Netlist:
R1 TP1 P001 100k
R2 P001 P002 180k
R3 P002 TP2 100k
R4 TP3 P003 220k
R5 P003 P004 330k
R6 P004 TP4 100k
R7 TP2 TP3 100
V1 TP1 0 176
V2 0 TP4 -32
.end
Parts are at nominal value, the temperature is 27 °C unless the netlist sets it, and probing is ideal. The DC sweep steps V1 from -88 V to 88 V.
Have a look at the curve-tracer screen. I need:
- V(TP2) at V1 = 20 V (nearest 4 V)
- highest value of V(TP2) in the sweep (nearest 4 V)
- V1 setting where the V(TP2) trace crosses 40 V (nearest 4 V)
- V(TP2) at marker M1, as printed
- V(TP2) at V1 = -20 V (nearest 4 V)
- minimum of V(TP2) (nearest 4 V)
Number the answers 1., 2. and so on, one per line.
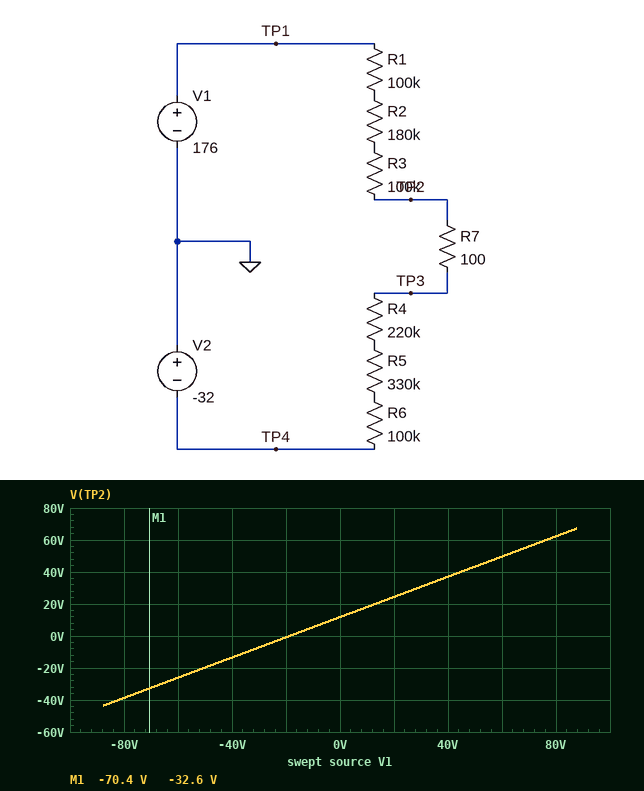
1. 24 V
2. 68 V
3. 44 V
4. -32.6 V
5. 0 V
6. -44 V
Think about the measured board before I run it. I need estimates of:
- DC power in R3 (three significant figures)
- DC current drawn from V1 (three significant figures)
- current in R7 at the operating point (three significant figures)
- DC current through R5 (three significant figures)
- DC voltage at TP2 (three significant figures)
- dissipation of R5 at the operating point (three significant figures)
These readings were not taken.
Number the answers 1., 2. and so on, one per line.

1. 1.95 mW
2. 140 µA
3. 140 µA
4. 140 µA
5. 123 V
6. 6.45 mW
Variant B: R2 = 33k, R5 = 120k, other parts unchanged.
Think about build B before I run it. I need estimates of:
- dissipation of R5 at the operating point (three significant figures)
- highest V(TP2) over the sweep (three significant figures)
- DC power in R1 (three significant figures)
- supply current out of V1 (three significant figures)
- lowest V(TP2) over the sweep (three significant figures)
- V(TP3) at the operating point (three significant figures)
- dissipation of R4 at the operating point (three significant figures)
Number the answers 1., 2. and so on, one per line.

1. 5.49 mW
2. 68.6 V
3. 4.58 mW
4. 214 µA
5. -46.5 V
6. 126 V
7. 10.1 mW
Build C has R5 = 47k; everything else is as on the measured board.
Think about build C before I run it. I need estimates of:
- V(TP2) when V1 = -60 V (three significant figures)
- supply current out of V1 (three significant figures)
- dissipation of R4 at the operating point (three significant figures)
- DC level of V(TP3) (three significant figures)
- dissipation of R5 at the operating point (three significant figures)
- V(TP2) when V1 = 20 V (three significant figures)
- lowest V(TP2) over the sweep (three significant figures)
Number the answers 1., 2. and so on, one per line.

1. -13.2 V
2. 193 µA
3. 8.17 mW
4. 103 V
5. 1.75 mW
6. 26.1 V
7. -27.0 V
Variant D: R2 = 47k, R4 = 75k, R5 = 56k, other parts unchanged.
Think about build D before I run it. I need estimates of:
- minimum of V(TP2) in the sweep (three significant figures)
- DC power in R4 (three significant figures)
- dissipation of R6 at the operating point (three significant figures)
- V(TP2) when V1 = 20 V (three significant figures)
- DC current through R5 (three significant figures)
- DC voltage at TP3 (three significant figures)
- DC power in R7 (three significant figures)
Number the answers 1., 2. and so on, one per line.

1. -26.0 V
2. 6.80 mW
3. 9.07 mW
4. 26.2 V
5. 301 µA
6. 102 V
7. 9.07 µW
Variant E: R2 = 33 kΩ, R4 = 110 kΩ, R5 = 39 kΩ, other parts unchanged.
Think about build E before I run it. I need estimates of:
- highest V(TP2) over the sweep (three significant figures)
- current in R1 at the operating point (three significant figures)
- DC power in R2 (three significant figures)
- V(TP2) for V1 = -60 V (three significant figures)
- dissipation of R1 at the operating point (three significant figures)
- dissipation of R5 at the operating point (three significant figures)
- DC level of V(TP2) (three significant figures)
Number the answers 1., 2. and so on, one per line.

1. 60.9 V
2. 299 µA
3. 2.94 mW
4. -15.5 V
5. 8.92 mW
6. 3.48 mW
7. 106 V
